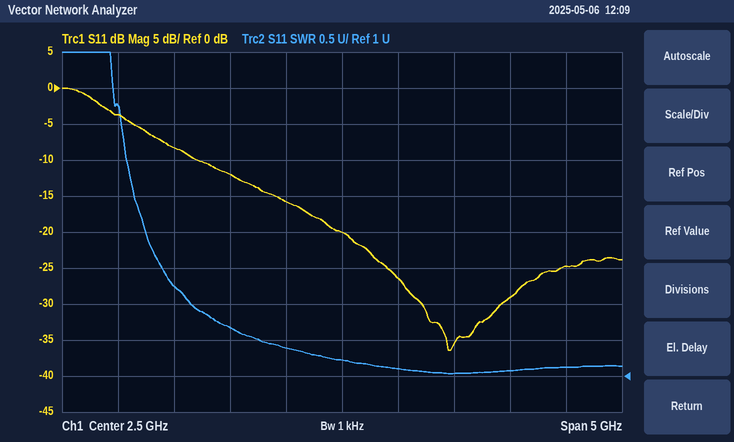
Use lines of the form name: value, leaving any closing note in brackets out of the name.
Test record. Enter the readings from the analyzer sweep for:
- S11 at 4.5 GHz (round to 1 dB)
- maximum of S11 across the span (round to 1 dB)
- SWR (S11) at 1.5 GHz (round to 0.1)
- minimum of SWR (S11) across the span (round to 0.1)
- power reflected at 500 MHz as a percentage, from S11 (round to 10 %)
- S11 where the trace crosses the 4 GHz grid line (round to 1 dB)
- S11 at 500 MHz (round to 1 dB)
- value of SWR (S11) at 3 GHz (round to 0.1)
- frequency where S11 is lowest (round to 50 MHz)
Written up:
S11 at 4.5 GHz: -25 dB
maximum of S11 across the span: 0 dB
SWR (S11) at 1.5 GHz: 1.7
minimum of SWR (S11) across the span: 1.0
power reflected at 500 MHz as a percentage, from S11: 40 %
S11 where the trace crosses the 4 GHz grid line: -29 dB
S11 at 500 MHz: -4 dB
value of SWR (S11) at 3 GHz: 1.1
frequency where S11 is lowest: 3.45 GHz
